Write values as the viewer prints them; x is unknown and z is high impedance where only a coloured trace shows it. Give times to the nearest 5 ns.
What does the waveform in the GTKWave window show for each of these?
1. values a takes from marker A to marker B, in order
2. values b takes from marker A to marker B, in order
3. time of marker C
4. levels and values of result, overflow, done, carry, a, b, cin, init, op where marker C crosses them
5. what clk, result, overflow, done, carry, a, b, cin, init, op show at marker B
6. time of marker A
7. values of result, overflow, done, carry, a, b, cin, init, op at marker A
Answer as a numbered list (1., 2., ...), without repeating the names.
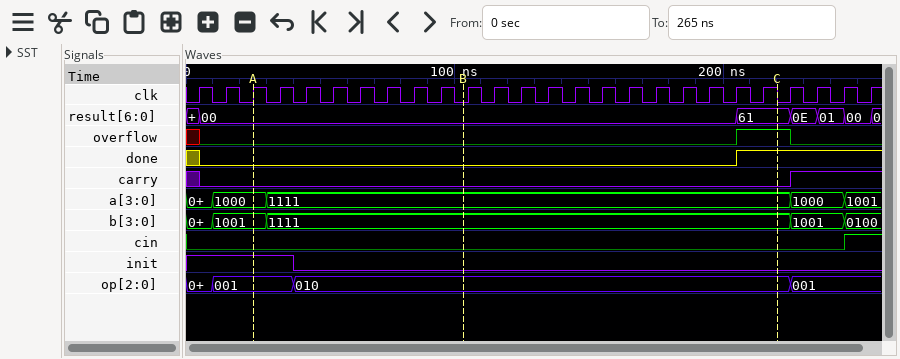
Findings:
1. 1000, 1111
2. 1001, 1111
3. 220 ns
4. result=61, overflow=1, done=1, carry=0, a=1111, b=1111, cin=0, init=0, op=010
5. clk=0, result=00, overflow=0, done=0, carry=0, a=1111, b=1111, cin=0, init=0, op=010
6. 25 ns
7. result=00, overflow=0, done=0, carry=0, a=1000, b=1001, cin=0, init=1, op=001
